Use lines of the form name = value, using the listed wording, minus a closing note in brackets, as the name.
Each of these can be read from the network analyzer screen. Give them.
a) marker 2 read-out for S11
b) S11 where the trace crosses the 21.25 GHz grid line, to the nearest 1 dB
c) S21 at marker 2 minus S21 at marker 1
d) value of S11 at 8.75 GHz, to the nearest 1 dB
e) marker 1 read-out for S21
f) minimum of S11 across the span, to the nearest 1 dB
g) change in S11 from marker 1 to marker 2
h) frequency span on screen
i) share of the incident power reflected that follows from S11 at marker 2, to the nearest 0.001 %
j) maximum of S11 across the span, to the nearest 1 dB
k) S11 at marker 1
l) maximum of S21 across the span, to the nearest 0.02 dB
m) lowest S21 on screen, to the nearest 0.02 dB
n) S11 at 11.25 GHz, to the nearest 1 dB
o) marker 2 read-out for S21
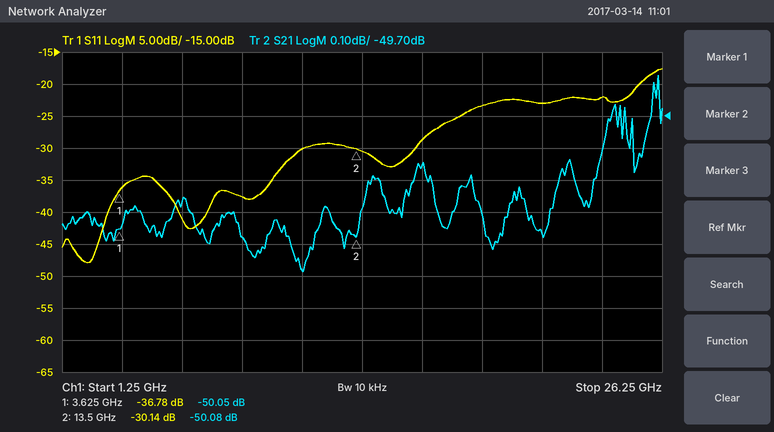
marker 2 read-out for S11 = -30.14 dB
S11 where the trace crosses the 21.25 GHz grid line, to the nearest 1 dB = -23 dB
S21 at marker 2 minus S21 at marker 1 = -0.03 dB
value of S11 at 8.75 GHz, to the nearest 1 dB = -38 dB
marker 1 read-out for S21 = -50.05 dB
minimum of S11 across the span, to the nearest 1 dB = -48 dB
change in S11 from marker 1 to marker 2 = 6.64 dB
frequency span on screen = 25 GHz
share of the incident power reflected that follows from S11 at marker 2, to the nearest 0.001 % = 0.097 %
maximum of S11 across the span, to the nearest 1 dB = -18 dB
S11 at marker 1 = -36.78 dB
maximum of S21 across the span, to the nearest 0.02 dB = -49.58 dB
lowest S21 on screen, to the nearest 0.02 dB = -50.18 dB
S11 at 11.25 GHz, to the nearest 1 dB = -30 dB
marker 2 read-out for S21 = -50.08 dB
